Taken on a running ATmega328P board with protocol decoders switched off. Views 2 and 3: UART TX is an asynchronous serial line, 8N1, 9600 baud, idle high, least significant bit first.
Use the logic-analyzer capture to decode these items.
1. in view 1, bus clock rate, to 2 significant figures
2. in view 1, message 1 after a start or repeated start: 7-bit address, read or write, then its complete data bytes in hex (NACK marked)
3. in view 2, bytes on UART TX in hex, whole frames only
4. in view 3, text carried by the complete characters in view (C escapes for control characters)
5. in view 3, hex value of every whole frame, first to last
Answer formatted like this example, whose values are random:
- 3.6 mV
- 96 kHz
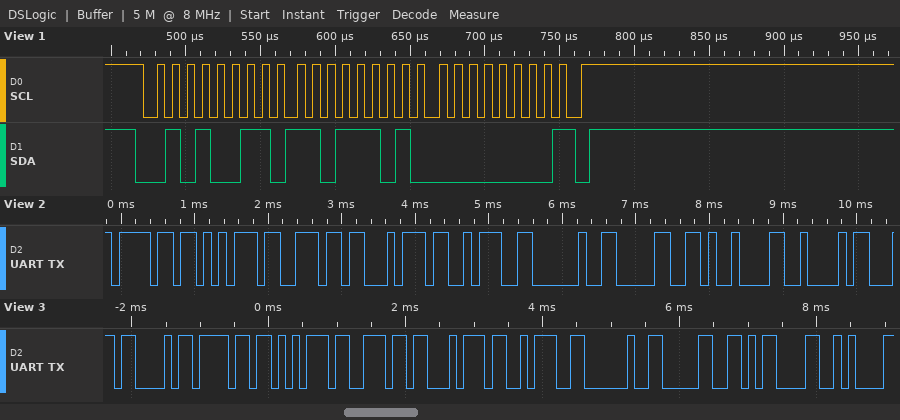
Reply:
- 100 kHz
- 0x29 read: DD 00 NACK
- 0x6F 0x75 0x6E 0x74 0x3A 0x20 0x30 0x09 0x42
- "Count: 0\r\n"
- 43 6F 75 6E 74 3A 20 30 0D 0A
